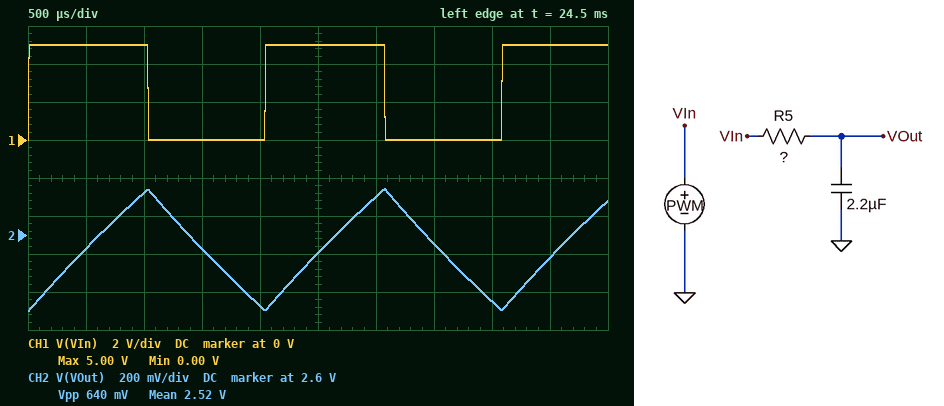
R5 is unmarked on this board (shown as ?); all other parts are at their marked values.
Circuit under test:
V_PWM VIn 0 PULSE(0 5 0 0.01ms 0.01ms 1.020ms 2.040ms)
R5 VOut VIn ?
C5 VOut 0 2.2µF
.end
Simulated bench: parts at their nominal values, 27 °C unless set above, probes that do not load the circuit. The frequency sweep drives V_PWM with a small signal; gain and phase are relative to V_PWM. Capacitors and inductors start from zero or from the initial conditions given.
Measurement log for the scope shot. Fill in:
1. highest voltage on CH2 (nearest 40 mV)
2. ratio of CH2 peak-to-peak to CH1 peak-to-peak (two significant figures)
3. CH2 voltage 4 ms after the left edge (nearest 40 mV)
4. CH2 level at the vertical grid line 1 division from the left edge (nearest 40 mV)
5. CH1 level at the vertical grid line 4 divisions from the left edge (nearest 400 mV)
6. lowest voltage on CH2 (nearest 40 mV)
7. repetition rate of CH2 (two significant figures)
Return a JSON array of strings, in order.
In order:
["2.84 V", "0.13", "2.24 V", "2.52 V", "0 V", "2.20 V", "490 Hz"]
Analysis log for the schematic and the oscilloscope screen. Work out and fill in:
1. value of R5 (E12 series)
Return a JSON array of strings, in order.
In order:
["1.8 kΩ"]
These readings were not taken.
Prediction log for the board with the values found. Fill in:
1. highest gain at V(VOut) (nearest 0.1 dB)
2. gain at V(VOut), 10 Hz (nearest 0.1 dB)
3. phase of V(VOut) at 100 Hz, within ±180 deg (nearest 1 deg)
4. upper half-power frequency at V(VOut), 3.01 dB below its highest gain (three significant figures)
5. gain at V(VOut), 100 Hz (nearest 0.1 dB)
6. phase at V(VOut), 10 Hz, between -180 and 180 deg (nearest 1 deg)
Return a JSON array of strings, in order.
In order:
["0 dB", "-0.3 dB", "-68 deg", "40.2 Hz", "-8.6 dB", "-14 deg"]
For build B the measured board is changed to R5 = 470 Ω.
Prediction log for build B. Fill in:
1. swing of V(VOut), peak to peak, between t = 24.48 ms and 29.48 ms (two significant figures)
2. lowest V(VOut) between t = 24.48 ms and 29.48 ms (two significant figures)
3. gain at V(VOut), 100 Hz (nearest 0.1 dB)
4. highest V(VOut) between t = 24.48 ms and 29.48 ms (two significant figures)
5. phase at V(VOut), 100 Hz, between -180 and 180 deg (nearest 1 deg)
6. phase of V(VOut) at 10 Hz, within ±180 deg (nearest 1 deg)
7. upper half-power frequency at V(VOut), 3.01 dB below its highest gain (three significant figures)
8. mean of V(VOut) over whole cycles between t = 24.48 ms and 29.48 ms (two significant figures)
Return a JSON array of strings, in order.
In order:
["2.3 V", "1.4 V", "-1.5 dB", "3.7 V", "-33 deg", "-4 deg", "154 Hz", "2.5 V"]
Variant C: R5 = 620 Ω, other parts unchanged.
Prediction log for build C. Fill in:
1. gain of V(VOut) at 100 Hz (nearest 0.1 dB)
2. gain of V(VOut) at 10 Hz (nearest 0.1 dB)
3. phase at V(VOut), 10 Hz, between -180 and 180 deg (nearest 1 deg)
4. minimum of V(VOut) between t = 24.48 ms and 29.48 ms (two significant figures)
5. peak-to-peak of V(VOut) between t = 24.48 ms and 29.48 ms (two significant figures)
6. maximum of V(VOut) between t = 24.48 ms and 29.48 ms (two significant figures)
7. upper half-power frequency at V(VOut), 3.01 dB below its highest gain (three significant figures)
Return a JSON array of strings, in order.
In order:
["-2.4 dB", "0 dB", "-5 deg", "1.6 V", "1.8 V", "3.4 V", "117 Hz"]
